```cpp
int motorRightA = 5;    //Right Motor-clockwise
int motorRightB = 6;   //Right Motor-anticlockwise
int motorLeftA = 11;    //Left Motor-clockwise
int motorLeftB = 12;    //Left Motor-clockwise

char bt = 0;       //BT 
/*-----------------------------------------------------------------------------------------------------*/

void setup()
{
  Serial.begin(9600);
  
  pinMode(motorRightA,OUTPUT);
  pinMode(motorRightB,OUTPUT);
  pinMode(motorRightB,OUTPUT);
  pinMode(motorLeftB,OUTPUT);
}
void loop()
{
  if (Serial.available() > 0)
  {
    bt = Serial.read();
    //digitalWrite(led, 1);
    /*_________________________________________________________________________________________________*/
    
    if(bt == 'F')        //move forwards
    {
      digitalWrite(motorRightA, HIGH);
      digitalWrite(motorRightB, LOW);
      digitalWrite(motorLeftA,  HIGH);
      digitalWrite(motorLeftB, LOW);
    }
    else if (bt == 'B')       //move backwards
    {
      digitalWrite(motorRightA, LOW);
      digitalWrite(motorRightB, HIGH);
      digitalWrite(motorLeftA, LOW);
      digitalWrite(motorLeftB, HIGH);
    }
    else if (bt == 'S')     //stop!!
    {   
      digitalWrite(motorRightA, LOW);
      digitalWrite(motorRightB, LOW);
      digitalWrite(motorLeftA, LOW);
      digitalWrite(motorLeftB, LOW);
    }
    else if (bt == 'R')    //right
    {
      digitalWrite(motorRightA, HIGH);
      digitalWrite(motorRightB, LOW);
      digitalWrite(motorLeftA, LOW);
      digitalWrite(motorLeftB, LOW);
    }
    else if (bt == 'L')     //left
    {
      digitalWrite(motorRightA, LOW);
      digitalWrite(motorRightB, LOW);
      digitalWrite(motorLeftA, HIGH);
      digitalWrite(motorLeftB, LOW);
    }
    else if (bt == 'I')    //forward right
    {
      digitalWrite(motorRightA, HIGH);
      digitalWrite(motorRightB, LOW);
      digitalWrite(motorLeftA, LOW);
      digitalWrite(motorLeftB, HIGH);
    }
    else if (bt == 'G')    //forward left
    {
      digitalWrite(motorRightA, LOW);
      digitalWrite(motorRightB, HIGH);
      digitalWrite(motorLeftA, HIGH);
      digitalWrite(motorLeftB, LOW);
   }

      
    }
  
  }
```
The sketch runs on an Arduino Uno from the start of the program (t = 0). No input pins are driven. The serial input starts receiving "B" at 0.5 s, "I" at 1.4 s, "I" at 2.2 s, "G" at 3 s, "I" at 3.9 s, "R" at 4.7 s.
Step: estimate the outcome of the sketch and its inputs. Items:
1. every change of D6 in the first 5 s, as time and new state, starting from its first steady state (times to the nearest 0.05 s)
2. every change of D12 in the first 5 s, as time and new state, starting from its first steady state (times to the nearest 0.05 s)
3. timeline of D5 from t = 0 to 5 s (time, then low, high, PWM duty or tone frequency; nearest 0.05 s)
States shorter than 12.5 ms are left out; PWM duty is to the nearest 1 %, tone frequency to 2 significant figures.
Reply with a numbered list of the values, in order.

1. 0 s low; 0.5 s high; 1.4 s low; 3 s high; 3.9 s low
2. 0 s low; 0.5 s high; 3 s low; 3.9 s high; 4.7 s low
3. 0 s low; 1.4 s high; 3 s low; 3.9 s high
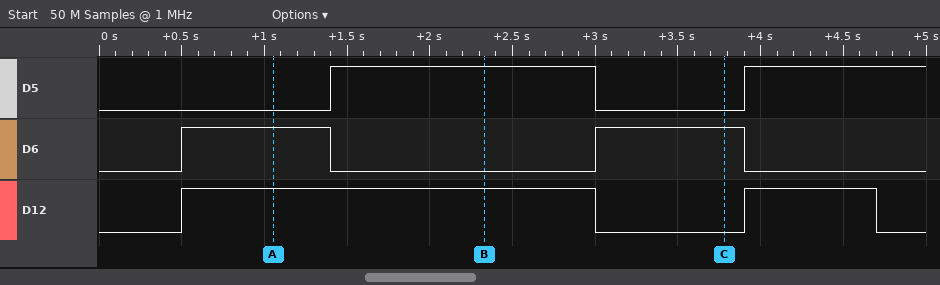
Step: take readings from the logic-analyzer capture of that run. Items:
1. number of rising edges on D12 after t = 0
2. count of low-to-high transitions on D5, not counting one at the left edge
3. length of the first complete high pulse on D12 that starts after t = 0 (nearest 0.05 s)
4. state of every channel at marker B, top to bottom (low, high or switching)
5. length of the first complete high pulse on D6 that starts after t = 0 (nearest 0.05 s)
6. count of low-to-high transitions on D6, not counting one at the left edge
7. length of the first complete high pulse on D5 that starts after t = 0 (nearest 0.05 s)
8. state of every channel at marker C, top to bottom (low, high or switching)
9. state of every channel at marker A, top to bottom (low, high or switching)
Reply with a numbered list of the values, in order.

1. 2
2. 2
3. 2.50 s
4. D5 high, D6 low, D12 high
5. 0.90 s
6. 2
7. 1.60 s
8. D5 low, D6 high, D12 low
9. D5 low, D6 high, D12 high
